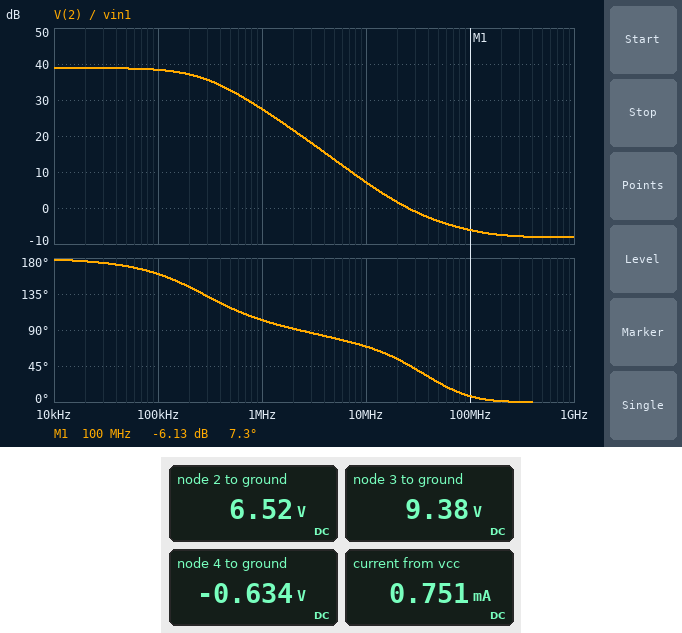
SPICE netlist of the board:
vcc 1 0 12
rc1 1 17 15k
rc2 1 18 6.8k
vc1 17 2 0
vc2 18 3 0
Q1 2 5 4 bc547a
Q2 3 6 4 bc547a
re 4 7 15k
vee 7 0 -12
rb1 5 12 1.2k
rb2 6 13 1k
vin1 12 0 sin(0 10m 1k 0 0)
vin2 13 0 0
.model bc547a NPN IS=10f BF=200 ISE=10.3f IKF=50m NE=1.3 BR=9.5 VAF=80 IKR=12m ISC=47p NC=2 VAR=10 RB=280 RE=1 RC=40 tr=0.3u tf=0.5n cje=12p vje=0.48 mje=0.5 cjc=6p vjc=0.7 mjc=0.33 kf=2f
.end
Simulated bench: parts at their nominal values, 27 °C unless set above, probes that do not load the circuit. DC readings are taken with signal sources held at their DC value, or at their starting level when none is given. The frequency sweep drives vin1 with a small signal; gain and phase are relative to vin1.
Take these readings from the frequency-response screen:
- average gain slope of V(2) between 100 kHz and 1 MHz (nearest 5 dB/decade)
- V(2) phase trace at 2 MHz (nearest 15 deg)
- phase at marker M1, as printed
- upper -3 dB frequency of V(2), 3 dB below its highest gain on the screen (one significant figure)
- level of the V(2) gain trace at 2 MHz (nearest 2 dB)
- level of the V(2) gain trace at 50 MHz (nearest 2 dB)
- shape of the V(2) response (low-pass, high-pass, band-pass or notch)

-10 dB/decade
90 deg
7.3 deg
300 kHz
22 dB
-4 dB
low-pass
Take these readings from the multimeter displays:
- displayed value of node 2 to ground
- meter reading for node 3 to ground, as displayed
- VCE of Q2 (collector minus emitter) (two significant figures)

6.52 V
9.38 V
10 V
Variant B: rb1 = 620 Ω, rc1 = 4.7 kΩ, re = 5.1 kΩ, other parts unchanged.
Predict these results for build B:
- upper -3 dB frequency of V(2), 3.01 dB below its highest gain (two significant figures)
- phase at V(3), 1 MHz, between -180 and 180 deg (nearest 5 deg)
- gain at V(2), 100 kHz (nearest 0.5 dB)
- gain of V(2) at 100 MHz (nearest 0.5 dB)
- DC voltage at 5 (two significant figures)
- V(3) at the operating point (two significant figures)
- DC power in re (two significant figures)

270 kHz
-75 deg
36.0 dB
-4.5 dB
-5.7 mV
4.9 V
25 mW
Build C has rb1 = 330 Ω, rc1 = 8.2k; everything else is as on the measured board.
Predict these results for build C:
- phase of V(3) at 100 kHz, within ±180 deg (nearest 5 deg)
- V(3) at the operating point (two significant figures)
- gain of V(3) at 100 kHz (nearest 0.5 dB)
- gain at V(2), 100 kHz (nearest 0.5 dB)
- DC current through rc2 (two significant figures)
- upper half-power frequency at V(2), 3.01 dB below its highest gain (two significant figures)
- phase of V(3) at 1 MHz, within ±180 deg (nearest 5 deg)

-10 deg
9.5 V
32.5 dB
34.0 dB
360 µA
600 kHz
-60 deg
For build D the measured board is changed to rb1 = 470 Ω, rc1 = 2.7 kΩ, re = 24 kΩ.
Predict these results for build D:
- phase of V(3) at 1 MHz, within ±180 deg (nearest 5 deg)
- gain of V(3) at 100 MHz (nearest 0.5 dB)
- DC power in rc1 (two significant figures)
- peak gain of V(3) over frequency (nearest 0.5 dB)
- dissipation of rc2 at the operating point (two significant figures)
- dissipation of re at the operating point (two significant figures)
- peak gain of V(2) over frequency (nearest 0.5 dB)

-45 deg
-8.5 dB
160 µW
29.0 dB
360 µW
5.4 mW
21.0 dB
